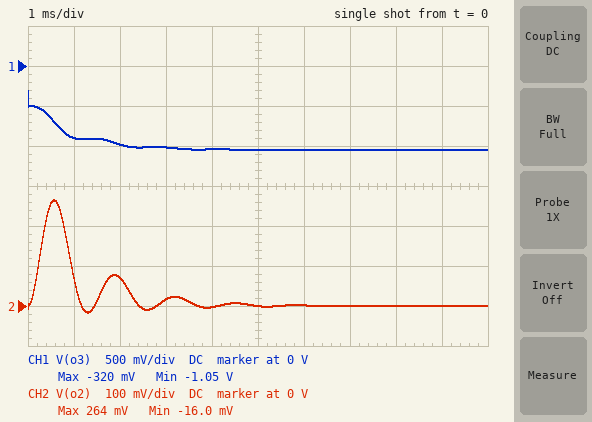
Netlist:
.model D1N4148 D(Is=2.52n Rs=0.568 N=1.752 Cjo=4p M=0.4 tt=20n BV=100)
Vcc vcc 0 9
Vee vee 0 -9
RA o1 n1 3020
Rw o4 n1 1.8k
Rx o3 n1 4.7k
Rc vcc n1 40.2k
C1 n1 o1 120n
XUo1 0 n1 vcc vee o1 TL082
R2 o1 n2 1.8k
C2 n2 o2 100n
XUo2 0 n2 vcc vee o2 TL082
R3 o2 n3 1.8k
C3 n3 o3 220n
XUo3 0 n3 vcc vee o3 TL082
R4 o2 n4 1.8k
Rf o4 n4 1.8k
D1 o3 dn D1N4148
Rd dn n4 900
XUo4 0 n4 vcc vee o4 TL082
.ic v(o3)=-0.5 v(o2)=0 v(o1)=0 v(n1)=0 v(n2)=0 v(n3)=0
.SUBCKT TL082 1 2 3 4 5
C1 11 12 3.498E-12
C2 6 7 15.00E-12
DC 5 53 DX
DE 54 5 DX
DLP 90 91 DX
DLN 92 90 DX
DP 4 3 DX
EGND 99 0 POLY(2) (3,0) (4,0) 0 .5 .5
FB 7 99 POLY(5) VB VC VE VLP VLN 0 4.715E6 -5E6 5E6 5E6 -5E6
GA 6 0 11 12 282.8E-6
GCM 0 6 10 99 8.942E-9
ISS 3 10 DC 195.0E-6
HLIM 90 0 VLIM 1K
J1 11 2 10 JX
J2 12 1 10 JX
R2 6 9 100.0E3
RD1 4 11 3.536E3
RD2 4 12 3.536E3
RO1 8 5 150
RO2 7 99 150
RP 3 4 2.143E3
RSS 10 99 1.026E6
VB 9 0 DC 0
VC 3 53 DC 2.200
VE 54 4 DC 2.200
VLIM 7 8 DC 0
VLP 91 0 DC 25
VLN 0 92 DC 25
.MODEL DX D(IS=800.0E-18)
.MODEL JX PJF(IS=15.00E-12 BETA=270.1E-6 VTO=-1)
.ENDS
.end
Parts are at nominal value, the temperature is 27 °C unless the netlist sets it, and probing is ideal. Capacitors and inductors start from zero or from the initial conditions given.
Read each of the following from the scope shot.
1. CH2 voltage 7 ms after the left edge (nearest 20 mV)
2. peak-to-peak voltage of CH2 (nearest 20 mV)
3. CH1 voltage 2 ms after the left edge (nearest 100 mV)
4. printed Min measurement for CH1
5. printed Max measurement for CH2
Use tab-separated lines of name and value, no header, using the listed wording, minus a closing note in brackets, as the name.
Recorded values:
CH2 voltage 7 ms after the left edge	0 V
peak-to-peak voltage of CH2	280 mV
CH1 voltage 2 ms after the left edge	-1.0 V
printed Min measurement for CH1	-1.05 V
printed Max measurement for CH2	264 mV
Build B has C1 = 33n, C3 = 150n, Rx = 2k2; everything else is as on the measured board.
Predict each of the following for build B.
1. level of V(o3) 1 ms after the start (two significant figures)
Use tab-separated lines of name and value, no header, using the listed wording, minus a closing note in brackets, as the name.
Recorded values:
level of V(o3) 1 ms after the start	-490 mV
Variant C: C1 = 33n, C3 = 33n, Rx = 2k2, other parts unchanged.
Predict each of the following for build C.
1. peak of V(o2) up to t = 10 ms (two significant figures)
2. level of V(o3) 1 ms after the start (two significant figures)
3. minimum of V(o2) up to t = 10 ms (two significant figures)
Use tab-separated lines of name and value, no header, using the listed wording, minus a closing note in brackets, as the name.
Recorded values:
peak of V(o2) up to t = 10 ms	730 mV
level of V(o3) 1 ms after the start	-480 mV
minimum of V(o2) up to t = 10 ms	-890 mV
